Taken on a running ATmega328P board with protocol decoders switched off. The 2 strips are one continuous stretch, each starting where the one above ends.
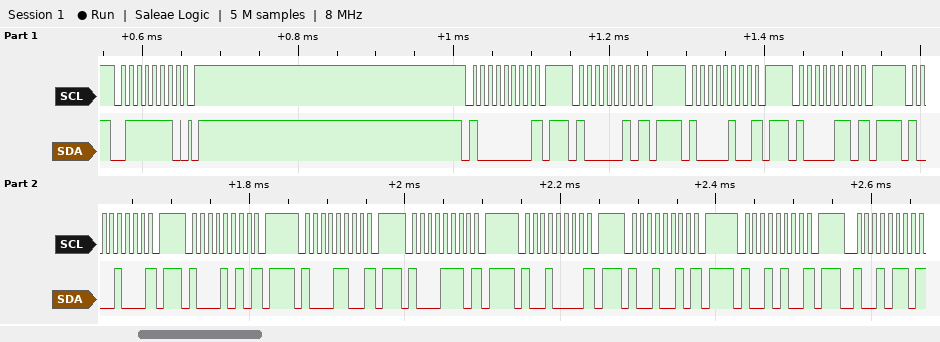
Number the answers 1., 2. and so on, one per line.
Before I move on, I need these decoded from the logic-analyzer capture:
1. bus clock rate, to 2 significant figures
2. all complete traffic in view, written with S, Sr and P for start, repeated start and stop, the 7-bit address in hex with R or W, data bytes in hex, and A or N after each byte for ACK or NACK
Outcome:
1. 100 kHz
2. S 3FW A P S 40W N P S 41W N P S 42W N P S 43W N P S 44W N P S 45W N P S 46W N P S 47W N P S 48W N P S 49W N P S 4AW N P S 4BW N
